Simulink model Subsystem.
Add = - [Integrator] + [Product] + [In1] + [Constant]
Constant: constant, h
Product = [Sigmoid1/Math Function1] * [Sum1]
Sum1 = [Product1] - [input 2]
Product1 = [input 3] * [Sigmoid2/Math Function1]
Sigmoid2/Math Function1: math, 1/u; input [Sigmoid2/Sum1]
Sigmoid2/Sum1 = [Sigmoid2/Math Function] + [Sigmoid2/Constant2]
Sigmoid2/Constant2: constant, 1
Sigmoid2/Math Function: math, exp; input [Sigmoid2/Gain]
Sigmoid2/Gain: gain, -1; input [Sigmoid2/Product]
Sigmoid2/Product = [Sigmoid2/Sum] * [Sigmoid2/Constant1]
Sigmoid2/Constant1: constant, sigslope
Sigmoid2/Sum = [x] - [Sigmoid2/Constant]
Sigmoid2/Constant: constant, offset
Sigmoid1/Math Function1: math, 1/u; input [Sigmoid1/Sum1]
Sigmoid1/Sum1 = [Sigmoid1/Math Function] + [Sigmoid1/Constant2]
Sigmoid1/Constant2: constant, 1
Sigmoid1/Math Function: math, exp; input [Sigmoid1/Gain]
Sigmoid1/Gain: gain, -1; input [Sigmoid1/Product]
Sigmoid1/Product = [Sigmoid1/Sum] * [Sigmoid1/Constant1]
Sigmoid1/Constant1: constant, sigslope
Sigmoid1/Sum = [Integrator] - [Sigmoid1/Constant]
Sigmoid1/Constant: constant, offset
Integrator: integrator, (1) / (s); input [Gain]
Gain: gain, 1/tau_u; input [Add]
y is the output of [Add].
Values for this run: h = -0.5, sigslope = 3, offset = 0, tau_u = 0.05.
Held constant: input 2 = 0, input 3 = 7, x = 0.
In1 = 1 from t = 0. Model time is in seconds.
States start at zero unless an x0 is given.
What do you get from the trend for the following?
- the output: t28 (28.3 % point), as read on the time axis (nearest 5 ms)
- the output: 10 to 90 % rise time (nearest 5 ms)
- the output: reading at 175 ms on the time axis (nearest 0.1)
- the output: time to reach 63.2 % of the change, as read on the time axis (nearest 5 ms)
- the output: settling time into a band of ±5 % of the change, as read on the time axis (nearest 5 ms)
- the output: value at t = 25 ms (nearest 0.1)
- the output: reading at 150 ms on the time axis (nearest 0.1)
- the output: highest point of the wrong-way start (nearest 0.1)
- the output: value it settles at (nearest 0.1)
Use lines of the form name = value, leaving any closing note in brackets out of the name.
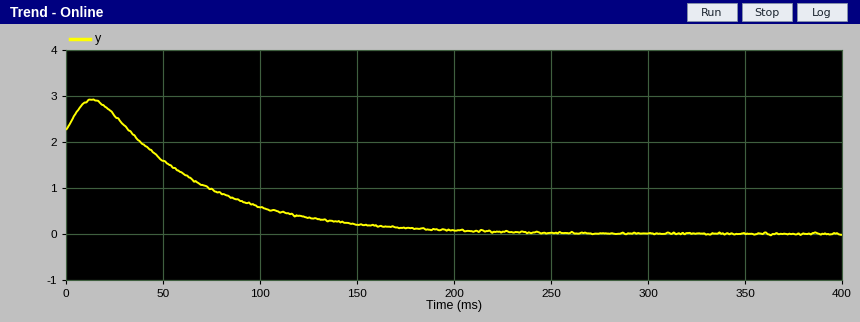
the output: t28 (28.3 % point), as read on the time axis = 50 ms
the output: 10 to 90 % rise time = 110 ms
the output: reading at 175 ms on the time axis = 0.1
the output: time to reach 63.2 % of the change, as read on the time axis = 85 ms
the output: settling time into a band of ±5 % of the change, as read on the time axis = 185 ms
the output: value at t = 25 ms = 2.6
the output: reading at 150 ms on the time axis = 0.2
the output: highest point of the wrong-way start = 2.9
the output: value it settles at = 0.0
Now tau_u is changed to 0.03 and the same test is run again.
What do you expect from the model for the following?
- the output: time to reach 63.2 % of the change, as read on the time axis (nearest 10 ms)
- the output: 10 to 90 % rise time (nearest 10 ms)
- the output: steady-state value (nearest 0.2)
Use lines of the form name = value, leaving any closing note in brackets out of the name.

the output: time to reach 63.2 % of the change, as read on the time axis = 50 ms
the output: 10 to 90 % rise time = 70 ms
the output: steady-state value = 0.0
